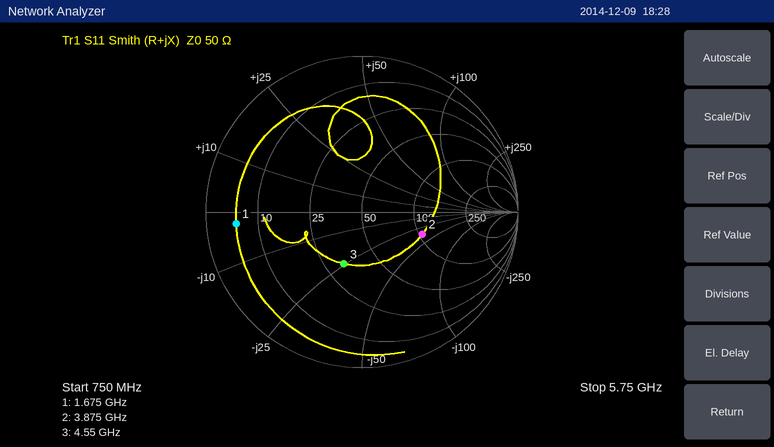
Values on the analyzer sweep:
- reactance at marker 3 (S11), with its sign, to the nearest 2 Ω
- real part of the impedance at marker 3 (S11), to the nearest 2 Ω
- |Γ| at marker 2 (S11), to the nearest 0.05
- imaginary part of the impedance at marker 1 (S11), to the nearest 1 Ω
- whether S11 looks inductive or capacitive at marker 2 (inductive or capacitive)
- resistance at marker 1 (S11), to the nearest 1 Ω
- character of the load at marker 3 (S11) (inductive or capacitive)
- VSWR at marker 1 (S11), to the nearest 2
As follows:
-24 Ω
32 Ω
0.40
-2 Ω
capacitive
5 Ω
capacitive
10
